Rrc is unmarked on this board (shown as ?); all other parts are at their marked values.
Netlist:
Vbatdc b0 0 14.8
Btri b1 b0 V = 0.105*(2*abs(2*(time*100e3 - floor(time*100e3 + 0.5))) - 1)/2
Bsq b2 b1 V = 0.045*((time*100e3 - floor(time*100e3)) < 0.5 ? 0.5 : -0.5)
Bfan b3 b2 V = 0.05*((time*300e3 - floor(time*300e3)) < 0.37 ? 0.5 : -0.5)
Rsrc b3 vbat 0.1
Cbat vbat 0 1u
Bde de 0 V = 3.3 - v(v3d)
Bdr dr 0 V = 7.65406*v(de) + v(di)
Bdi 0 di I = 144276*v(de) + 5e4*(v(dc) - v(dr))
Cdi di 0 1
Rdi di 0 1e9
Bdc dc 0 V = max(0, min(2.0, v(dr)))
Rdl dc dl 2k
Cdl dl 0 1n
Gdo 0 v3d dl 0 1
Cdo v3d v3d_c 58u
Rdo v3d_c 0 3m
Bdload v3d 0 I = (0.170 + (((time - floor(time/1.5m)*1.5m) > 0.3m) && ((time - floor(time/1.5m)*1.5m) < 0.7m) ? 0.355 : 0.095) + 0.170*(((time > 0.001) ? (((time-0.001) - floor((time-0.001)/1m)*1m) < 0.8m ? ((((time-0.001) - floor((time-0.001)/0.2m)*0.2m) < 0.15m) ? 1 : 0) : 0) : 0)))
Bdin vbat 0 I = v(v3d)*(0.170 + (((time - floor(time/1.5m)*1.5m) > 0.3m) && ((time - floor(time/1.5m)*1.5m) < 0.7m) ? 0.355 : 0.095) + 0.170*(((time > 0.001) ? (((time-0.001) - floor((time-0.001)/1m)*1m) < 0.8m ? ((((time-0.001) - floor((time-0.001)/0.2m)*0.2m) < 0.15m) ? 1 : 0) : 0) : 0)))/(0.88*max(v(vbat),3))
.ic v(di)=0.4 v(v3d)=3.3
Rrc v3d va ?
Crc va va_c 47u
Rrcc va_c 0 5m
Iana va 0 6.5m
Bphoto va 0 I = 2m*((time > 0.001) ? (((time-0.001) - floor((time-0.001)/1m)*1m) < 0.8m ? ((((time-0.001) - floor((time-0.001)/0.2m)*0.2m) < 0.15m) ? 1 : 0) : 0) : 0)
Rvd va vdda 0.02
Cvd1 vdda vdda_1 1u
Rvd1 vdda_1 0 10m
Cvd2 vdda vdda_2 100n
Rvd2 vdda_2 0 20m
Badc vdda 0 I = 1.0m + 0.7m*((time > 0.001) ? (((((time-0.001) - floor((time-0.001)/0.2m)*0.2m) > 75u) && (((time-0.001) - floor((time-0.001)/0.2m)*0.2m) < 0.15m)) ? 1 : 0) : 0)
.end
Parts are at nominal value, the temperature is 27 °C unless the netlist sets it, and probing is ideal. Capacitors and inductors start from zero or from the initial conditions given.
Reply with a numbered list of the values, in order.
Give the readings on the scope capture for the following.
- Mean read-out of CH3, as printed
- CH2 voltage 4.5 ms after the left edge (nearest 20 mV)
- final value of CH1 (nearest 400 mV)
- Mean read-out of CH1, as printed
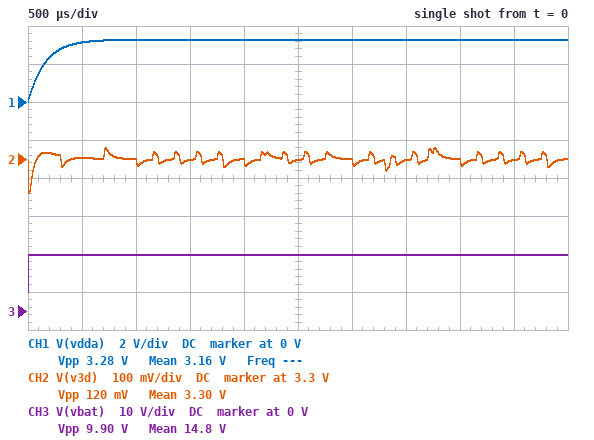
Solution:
1. 14.8 V
2. 3.30 V
3. 3.2 V
4. 3.16 V
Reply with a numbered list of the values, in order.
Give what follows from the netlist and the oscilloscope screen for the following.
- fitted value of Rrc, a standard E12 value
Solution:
1. 3.3 Ω
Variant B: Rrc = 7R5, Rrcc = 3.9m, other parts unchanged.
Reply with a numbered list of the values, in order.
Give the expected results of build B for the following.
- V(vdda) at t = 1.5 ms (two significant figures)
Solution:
1. 3.2 V
